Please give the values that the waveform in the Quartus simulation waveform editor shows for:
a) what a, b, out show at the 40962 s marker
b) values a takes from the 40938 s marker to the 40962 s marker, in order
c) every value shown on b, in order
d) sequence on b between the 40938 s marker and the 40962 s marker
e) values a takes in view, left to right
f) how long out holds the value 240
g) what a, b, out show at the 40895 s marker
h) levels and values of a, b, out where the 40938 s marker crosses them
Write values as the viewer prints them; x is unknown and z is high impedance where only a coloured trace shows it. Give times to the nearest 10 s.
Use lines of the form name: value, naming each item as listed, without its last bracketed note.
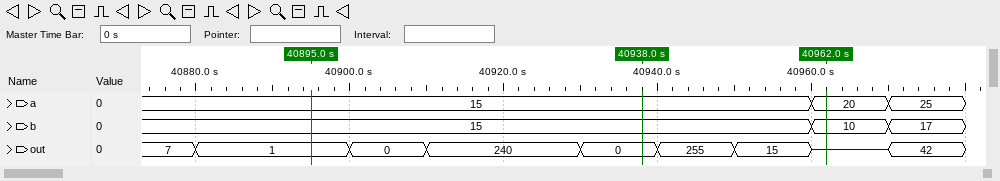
what a, b, out show at the 40962 s marker: a=20, b=10, out=z
values a takes from the 40938 s marker to the 40962 s marker, in order: 15, 20
every value shown on b, in order: 15, 10, 17
sequence on b between the 40938 s marker and the 40962 s marker: 15, 10
values a takes in view, left to right: 15, 20, 25
how long out holds the value 240: 20 s
what a, b, out show at the 40895 s marker: a=15, b=15, out=1
levels and values of a, b, out where the 40938 s marker crosses them: a=15, b=15, out=0
